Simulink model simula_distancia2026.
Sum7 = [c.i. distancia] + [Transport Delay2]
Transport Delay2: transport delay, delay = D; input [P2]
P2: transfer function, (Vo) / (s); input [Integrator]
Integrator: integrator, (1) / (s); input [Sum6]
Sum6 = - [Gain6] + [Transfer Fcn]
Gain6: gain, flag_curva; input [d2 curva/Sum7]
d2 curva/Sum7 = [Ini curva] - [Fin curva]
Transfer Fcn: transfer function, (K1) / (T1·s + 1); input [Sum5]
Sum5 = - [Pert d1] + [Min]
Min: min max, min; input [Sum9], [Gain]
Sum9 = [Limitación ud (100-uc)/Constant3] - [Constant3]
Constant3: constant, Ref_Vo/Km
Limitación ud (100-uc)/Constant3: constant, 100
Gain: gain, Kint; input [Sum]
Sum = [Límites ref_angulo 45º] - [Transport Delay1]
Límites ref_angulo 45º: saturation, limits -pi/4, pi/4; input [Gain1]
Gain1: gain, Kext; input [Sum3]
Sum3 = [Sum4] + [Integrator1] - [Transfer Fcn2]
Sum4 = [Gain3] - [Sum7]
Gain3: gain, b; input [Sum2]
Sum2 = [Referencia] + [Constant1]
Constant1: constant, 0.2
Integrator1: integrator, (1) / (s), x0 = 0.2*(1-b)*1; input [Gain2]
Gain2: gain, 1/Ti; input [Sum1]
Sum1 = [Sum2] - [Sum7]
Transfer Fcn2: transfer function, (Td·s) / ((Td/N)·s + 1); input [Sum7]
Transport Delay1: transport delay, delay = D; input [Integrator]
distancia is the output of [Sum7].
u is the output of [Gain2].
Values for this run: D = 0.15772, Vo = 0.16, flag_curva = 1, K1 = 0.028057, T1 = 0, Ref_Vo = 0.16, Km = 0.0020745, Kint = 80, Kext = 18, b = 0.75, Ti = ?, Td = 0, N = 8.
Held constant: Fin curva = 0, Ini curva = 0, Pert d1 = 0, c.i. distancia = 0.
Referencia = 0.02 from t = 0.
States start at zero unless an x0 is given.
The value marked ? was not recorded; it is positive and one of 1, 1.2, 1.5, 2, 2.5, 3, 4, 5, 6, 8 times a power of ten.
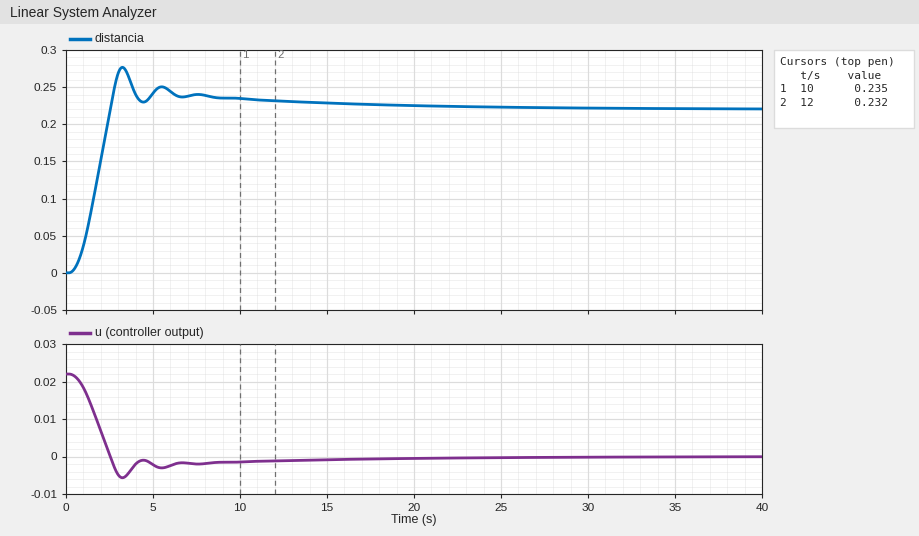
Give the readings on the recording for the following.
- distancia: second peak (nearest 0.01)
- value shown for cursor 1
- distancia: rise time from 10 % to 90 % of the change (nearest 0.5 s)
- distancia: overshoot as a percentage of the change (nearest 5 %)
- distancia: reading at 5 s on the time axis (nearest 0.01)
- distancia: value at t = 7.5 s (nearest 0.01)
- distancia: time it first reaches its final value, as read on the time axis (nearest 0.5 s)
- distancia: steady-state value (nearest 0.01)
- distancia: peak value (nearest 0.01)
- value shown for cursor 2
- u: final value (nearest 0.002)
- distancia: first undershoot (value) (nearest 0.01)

0.25
0.235
1.5 s
25 %
0.24
0.24
2.5 s
0.22
0.28
0.232
0.000
0.23
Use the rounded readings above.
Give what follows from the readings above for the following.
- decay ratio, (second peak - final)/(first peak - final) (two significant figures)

0.50
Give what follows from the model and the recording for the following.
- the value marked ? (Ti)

10
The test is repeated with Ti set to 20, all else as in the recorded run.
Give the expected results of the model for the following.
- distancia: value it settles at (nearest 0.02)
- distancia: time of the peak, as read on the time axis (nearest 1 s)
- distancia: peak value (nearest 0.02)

0.22
3 s
0.26
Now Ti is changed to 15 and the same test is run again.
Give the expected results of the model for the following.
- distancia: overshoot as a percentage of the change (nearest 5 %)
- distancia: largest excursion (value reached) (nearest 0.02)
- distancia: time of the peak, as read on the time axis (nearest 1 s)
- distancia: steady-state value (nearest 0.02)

20 %
0.26
3 s
0.22
